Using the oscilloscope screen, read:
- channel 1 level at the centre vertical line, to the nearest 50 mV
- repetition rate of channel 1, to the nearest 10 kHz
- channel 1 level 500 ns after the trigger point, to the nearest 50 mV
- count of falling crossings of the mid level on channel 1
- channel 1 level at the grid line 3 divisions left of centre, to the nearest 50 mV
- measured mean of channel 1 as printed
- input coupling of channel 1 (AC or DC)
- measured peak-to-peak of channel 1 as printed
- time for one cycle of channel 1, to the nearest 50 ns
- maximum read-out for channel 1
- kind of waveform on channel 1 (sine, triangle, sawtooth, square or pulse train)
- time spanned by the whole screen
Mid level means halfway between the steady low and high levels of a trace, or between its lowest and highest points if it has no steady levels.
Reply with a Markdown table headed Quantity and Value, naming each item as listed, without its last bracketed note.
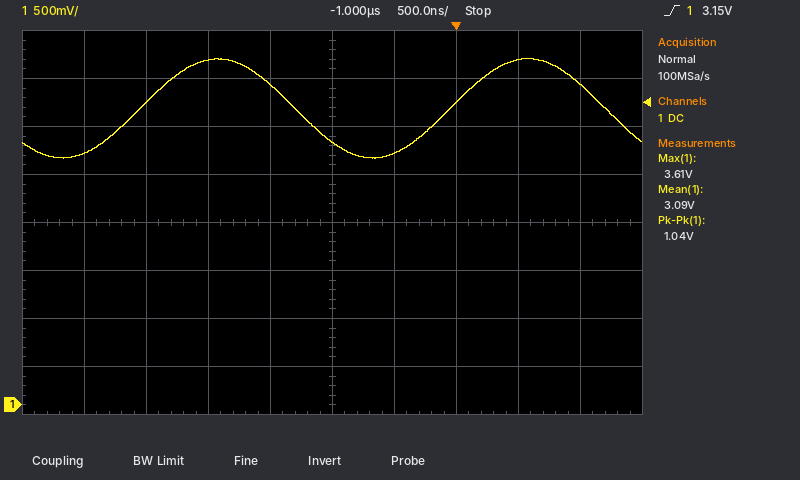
| Quantity | Value |
|---|---|
| channel 1 level at the centre vertical line, to the nearest 50 mV | 2.75 V |
| repetition rate of channel 1, to the nearest 10 kHz | 400 kHz |
| channel 1 level 500 ns after the trigger point, to the nearest 50 mV | 3.60 V |
| count of falling crossings of the mid level on channel 1 | 2 |
| channel 1 level at the grid line 3 divisions left of centre, to the nearest 50 mV | 3.15 V |
| measured mean of channel 1 as printed | 3.09 V |
| input coupling of channel 1 | DC |
| measured peak-to-peak of channel 1 as printed | 1.04 V |
| time for one cycle of channel 1, to the nearest 50 ns | 2.50 µs |
| maximum read-out for channel 1 | 3.61 V |
| kind of waveform on channel 1 | sine |
| time spanned by the whole screen | 5 µs |
